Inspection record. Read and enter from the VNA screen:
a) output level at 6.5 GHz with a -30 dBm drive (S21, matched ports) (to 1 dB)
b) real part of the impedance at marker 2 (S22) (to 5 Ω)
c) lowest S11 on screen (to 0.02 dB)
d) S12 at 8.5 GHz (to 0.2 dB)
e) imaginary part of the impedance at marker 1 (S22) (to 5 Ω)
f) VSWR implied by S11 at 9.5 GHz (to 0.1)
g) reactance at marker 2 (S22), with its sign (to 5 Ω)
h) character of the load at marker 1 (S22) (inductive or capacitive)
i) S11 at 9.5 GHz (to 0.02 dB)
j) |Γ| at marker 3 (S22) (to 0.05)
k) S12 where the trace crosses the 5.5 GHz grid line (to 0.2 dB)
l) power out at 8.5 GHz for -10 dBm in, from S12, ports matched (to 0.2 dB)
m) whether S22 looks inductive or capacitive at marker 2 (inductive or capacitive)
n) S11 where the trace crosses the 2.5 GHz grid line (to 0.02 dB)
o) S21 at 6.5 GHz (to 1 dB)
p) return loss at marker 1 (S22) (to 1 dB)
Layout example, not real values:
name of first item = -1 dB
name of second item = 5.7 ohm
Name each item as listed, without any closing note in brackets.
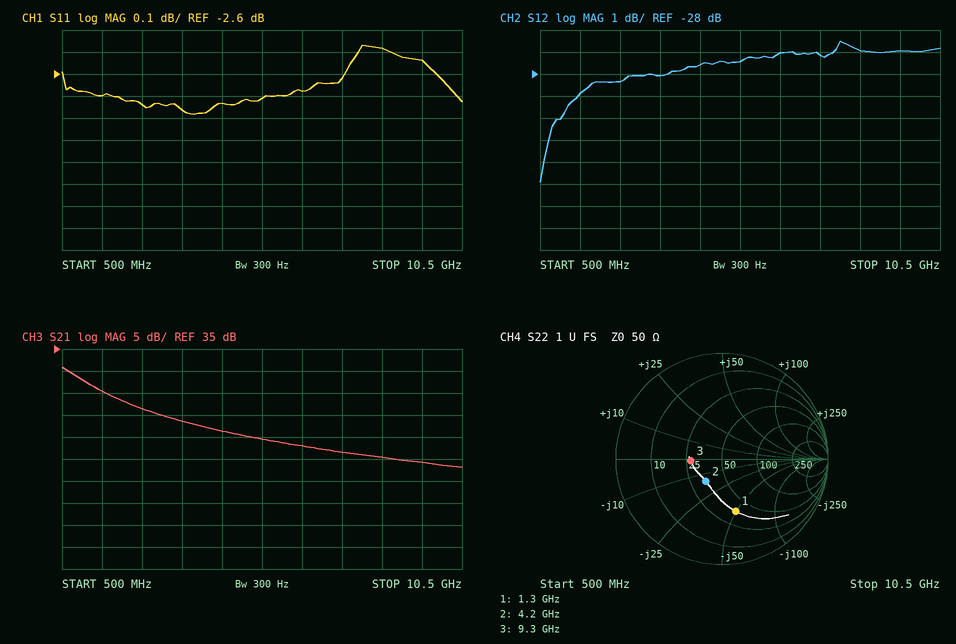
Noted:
output level at 6.5 GHz with a -30 dBm drive (S21, matched ports) = -17 dBm
real part of the impedance at marker 2 (S22) = 35 Ω
lowest S11 on screen = -2.78 dB
S12 at 8.5 GHz = -27.0 dB
imaginary part of the impedance at marker 1 (S22) = -50 Ω
VSWR implied by S11 at 9.5 GHz = 6.9
reactance at marker 2 (S22), with its sign = -15 Ω
character of the load at marker 1 (S22) = capacitive
S11 at 9.5 GHz = -2.54 dB
|Γ| at marker 3 (S22) = 0.30
S12 where the trace crosses the 5.5 GHz grid line = -27.4 dB
power out at 8.5 GHz for -10 dBm in, from S12, ports matched = -37.0 dBm
whether S22 looks inductive or capacitive at marker 2 = capacitive
S11 where the trace crosses the 2.5 GHz grid line = -2.74 dB
S21 at 6.5 GHz = 13 dB
return loss at marker 1 (S22) = 6 dB
